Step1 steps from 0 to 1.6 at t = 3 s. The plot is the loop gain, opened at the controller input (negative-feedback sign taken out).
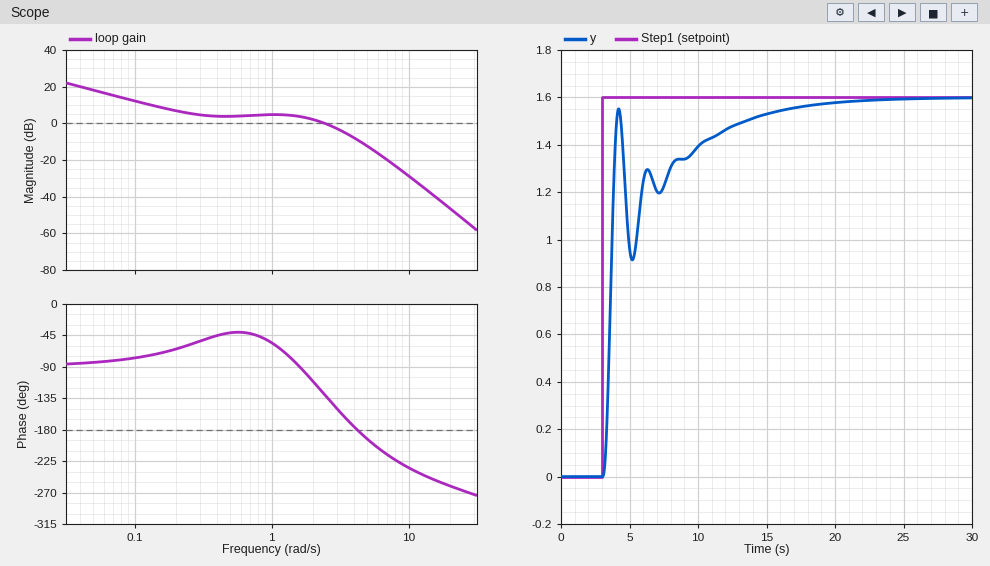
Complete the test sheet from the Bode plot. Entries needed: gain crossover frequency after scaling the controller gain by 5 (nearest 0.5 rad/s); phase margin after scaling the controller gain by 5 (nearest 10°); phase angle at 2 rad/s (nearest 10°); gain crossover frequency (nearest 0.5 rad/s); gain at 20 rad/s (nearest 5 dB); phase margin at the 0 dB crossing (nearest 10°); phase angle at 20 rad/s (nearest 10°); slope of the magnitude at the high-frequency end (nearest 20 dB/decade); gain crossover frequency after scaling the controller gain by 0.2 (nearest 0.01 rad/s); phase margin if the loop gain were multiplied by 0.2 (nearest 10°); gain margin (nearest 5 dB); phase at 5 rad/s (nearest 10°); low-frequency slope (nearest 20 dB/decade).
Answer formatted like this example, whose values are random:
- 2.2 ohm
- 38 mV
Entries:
- 5.5 rad/s
- -20°
- -110°
- 2.5 rad/s
- -45 dB
- 50°
- -260°
- -60 dB/decade
- 0.08 rad/s
- 100°
- 10 dB
- -190°
- -20 dB/decade
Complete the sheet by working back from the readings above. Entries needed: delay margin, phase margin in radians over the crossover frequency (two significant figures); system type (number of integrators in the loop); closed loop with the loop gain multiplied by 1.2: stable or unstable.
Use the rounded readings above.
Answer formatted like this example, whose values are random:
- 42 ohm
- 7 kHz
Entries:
- 0.35 s
- 1
- stable
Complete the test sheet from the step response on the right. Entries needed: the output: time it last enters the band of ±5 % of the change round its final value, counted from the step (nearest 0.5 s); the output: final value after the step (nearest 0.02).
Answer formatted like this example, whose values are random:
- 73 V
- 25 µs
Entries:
- 11.5 s
- 1.60
